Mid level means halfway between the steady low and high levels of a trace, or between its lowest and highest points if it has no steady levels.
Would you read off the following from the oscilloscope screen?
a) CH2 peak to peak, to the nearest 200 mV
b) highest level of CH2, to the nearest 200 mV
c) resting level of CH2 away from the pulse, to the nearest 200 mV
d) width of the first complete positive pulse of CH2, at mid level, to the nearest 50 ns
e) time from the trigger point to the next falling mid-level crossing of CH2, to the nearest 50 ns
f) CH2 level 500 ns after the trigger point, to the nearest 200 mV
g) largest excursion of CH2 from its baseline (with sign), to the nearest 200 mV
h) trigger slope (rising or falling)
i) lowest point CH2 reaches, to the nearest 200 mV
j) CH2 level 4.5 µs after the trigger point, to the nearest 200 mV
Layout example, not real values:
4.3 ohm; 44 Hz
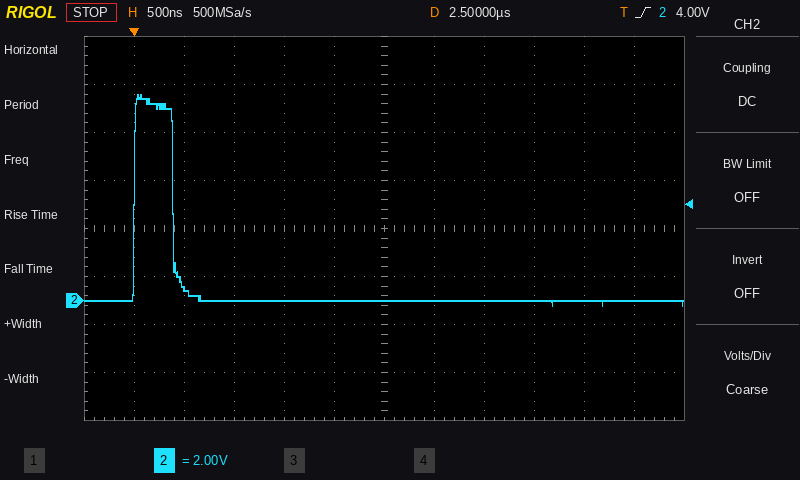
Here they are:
8.8 V; 8.6 V; 0.0 V; 400 ns; 400 ns; 600 mV; +8.6 V; rising; -200 mV; 0.0 V
